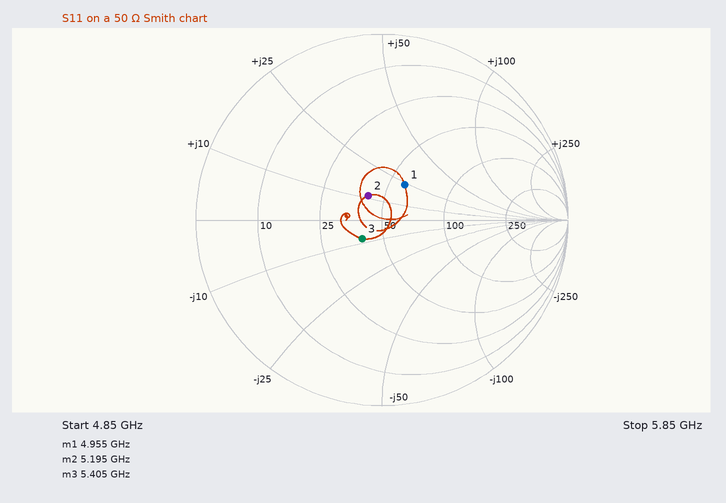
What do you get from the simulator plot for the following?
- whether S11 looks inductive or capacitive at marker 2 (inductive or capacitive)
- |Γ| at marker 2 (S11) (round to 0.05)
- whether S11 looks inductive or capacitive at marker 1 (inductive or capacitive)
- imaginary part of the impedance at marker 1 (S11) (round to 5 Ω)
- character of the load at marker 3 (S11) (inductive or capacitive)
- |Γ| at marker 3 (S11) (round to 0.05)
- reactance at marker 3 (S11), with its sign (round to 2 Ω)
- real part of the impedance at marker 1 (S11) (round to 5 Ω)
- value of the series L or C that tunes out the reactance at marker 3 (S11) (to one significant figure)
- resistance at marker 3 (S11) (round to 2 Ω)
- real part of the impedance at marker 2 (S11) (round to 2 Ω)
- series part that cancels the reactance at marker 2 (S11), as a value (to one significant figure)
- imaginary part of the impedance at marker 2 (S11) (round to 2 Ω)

inductive
0.15
inductive
+25 Ω
capacitive
0.15
-8 Ω
60 Ω
200 pH
40 Ω
42 Ω
3 pF
+12 Ω
